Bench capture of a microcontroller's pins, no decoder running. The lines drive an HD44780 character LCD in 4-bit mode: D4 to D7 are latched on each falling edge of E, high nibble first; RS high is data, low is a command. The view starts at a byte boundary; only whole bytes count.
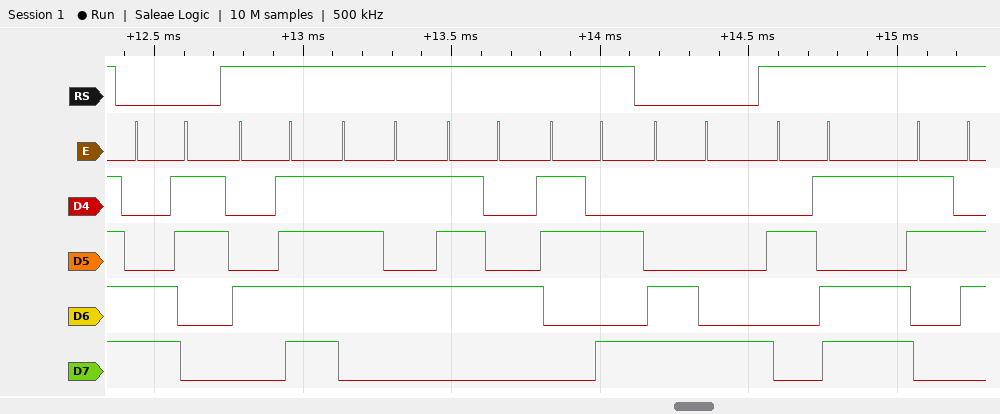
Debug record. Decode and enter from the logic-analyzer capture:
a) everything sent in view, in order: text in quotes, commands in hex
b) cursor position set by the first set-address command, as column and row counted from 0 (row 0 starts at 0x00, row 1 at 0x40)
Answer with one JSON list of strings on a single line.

["0xC3 \"Out:\" 0xC8 \"-6\"", "column 3, row 1"]
